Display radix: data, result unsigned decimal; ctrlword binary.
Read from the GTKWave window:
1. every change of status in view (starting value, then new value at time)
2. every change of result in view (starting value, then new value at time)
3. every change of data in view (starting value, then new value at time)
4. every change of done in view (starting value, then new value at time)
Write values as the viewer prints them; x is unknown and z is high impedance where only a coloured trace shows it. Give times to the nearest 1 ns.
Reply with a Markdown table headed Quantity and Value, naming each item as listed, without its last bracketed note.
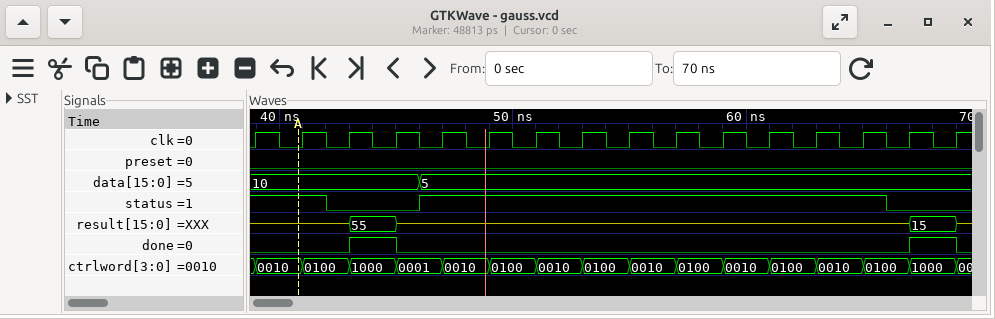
| Quantity | Value |
|---|---|
| every change of status in view | 1, 0 at 42 ns, 1 at 46 ns, 0 at 66 ns |
| every change of result in view | z, 55 at 43 ns, z at 45 ns, 15 at 67 ns, z at 69 ns |
| every change of data in view | 10, 5 at 46 ns |
| every change of done in view | 0, 1 at 43 ns, 0 at 45 ns, 1 at 67 ns, 0 at 69 ns |
